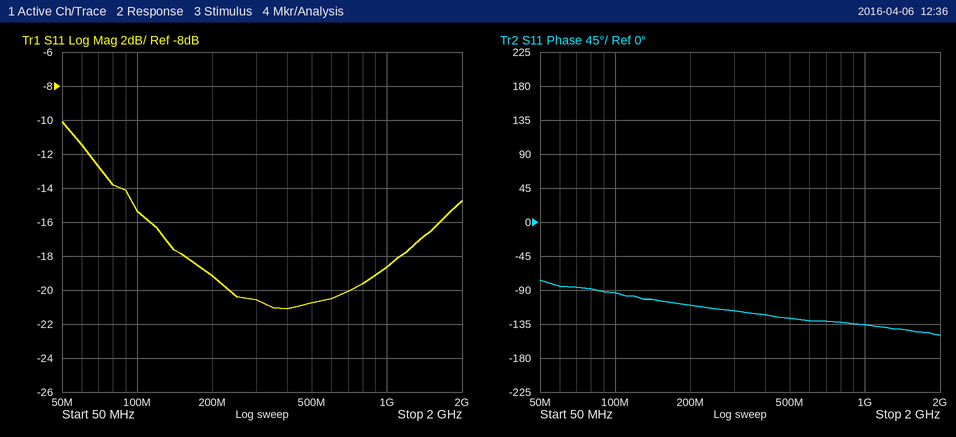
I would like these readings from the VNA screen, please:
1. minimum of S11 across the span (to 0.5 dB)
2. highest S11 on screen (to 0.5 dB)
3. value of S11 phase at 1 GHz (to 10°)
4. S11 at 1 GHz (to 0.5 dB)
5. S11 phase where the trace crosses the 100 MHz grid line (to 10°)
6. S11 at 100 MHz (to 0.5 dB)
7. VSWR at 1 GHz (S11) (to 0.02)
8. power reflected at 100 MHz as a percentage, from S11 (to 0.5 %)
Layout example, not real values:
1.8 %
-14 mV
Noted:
-21.0 dB
-10.0 dB
-140°
-18.5 dB
-90°
-15.5 dB
1.26
3.0 %
